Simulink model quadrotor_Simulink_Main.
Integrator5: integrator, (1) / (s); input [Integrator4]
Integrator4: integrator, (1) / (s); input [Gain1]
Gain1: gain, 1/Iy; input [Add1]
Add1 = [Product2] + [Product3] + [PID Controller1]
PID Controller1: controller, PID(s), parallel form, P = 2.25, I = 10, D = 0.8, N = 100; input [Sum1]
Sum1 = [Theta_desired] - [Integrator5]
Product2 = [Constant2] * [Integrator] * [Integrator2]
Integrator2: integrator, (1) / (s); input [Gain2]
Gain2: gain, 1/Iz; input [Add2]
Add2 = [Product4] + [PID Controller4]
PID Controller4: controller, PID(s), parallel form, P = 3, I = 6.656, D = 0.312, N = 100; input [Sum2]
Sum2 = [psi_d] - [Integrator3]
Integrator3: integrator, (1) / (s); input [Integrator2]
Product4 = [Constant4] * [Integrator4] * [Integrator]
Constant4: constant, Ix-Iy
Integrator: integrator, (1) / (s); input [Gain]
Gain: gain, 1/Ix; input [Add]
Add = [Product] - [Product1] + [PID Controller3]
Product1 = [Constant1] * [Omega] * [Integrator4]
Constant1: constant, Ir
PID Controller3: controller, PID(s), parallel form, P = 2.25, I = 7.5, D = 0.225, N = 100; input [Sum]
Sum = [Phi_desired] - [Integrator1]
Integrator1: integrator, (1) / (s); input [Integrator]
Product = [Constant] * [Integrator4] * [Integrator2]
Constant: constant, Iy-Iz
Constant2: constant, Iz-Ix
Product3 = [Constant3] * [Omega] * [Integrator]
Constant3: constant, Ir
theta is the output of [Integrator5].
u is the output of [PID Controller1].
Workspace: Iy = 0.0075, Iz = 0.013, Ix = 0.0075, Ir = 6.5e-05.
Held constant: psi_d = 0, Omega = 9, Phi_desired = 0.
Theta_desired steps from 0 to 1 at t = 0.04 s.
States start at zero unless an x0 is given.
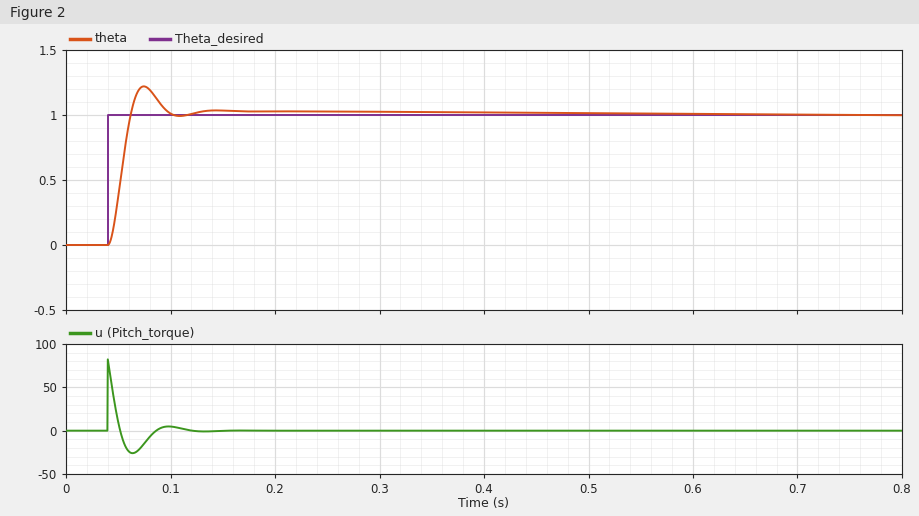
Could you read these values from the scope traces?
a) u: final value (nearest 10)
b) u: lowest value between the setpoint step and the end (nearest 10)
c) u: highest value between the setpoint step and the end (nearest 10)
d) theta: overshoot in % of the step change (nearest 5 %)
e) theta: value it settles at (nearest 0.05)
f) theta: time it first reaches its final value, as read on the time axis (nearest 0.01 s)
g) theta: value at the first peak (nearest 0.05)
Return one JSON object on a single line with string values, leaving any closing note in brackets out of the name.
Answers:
{"u: final value": "0", "u: lowest value between the setpoint step and the end": "-30", "u: highest value between the setpoint step and the end": "80", "theta: overshoot in % of the step change": "20 %", "theta: value it settles at": "1.00", "theta: time it first reaches its final value, as read on the time axis": "0.06 s", "theta: value at the first peak": "1.20"}
